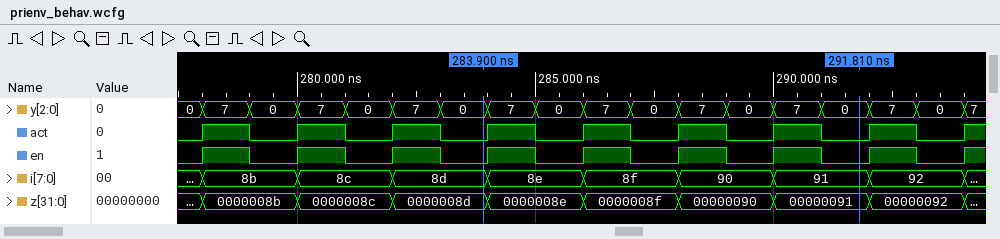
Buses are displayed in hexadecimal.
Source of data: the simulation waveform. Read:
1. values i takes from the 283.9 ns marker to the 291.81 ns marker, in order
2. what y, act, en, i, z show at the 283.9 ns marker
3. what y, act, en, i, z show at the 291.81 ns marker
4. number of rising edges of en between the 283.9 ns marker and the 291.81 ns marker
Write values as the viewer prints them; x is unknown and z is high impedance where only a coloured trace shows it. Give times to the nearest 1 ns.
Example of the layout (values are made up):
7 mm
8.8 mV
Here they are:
8d, 8e, 8f, 90, 91
y=0, act=0, en=0, i=8d, z=0000008d
y=0, act=0, en=0, i=91, z=00000091
4
